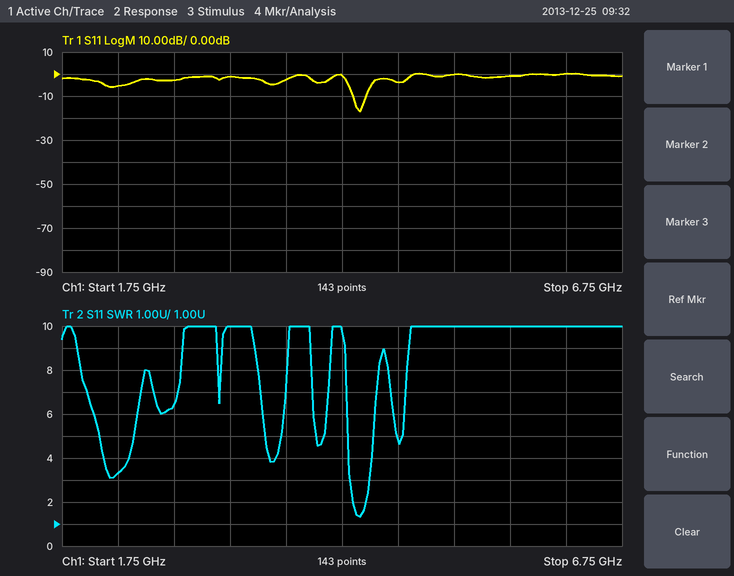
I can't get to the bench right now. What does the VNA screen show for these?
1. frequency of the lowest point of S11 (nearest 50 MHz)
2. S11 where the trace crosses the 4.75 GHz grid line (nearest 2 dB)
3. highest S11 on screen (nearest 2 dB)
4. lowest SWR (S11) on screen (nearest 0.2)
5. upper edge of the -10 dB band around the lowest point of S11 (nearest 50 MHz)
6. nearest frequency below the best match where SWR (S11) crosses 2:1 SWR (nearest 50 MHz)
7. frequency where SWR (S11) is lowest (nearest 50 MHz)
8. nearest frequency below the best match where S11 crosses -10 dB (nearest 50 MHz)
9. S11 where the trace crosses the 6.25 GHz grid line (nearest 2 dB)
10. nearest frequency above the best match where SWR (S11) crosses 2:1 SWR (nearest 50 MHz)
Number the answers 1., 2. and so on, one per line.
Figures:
1. 4.40 GHz
2. -4 dB
3. 0 dB
4. 1.4
5. 4.45 GHz
6. 4.35 GHz
7. 4.40 GHz
8. 4.35 GHz
9. 0 dB
10. 4.45 GHz
